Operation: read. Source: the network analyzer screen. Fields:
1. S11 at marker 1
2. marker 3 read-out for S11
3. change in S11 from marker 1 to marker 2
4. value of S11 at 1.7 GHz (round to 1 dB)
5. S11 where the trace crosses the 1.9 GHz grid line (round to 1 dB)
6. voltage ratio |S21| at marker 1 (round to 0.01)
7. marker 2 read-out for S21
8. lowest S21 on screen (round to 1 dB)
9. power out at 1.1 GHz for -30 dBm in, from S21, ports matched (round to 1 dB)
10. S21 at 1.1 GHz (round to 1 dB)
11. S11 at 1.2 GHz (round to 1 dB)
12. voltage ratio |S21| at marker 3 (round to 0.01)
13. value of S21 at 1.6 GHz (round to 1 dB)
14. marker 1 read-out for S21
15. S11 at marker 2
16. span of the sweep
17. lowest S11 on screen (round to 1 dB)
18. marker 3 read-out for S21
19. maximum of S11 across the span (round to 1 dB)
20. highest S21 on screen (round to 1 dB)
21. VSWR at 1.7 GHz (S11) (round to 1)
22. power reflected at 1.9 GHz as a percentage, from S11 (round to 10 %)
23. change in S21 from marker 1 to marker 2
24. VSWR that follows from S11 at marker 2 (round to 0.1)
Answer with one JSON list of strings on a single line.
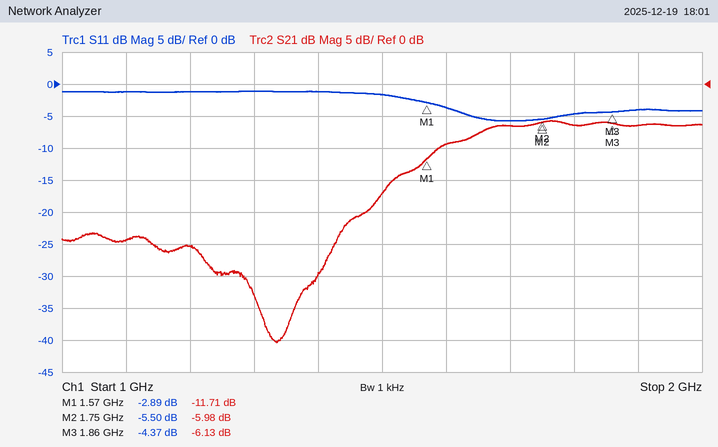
["-2.89 dB", "-4.37 dB", "-2.61 dB", "-6 dB", "-4 dB", "0.26", "-5.98 dB", "-40 dB", "-54 dBm", "-24 dB", "-1 dB", "0.49", "-9 dB", "-11.71 dB", "-5.50 dB", "1 GHz", "-6 dB", "-6.13 dB", "-1 dB", "-6 dB", "3", "40 %", "5.73 dB", "3.3"]
